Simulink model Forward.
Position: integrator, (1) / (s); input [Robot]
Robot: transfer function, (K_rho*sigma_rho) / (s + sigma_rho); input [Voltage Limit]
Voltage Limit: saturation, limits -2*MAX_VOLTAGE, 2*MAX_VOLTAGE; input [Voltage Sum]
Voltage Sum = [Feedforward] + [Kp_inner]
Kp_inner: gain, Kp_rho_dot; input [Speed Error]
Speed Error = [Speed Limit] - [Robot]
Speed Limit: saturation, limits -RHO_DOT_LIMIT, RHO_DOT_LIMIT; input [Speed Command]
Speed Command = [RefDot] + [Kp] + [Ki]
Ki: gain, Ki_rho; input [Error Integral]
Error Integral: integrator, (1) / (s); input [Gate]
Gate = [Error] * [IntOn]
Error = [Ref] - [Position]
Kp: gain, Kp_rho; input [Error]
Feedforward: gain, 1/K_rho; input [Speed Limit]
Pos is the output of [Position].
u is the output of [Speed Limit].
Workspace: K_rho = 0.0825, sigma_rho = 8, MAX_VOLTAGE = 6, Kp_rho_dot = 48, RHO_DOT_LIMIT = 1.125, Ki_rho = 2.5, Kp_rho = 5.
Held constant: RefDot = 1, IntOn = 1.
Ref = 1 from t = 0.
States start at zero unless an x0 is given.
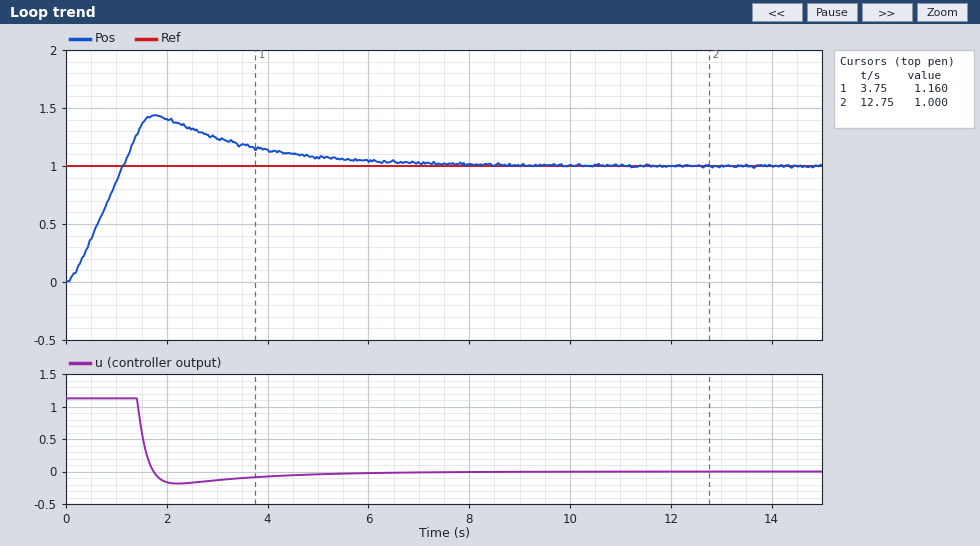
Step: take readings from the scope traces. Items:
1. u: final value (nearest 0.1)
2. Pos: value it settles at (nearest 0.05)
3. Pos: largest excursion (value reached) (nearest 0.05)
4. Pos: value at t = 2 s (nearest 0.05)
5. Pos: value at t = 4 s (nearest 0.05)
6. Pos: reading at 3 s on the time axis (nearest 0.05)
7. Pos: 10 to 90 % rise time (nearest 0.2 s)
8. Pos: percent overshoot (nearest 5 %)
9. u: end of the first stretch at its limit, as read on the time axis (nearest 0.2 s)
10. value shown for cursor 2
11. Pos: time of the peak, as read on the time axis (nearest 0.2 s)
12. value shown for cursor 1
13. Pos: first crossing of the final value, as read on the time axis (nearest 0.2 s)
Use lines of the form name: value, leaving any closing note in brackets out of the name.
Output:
u: final value: 0.0
Pos: value it settles at: 1.00
Pos: largest excursion (value reached): 1.45
Pos: value at t = 2 s: 1.40
Pos: value at t = 4 s: 1.15
Pos: reading at 3 s on the time axis: 1.25
Pos: 10 to 90 % rise time: 0.8 s
Pos: percent overshoot: 45 %
u: end of the first stretch at its limit, as read on the time axis: 1.4 s
value shown for cursor 2: 1.000
Pos: time of the peak, as read on the time axis: 1.8 s
value shown for cursor 1: 1.160
Pos: first crossing of the final value, as read on the time axis: 1.2 s
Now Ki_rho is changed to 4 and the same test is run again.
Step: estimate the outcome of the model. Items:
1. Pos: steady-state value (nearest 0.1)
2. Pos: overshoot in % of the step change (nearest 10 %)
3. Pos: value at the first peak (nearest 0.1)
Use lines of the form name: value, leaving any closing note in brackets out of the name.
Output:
Pos: steady-state value: 1.0
Pos: overshoot in % of the step change: 50 %
Pos: value at the first peak: 1.5
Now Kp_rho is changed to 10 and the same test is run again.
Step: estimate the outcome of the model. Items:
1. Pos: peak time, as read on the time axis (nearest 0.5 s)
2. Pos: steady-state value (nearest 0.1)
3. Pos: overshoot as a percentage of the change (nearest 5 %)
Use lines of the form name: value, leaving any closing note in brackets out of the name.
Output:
Pos: peak time, as read on the time axis: 1.5 s
Pos: steady-state value: 1.0
Pos: overshoot as a percentage of the change: 25 %
